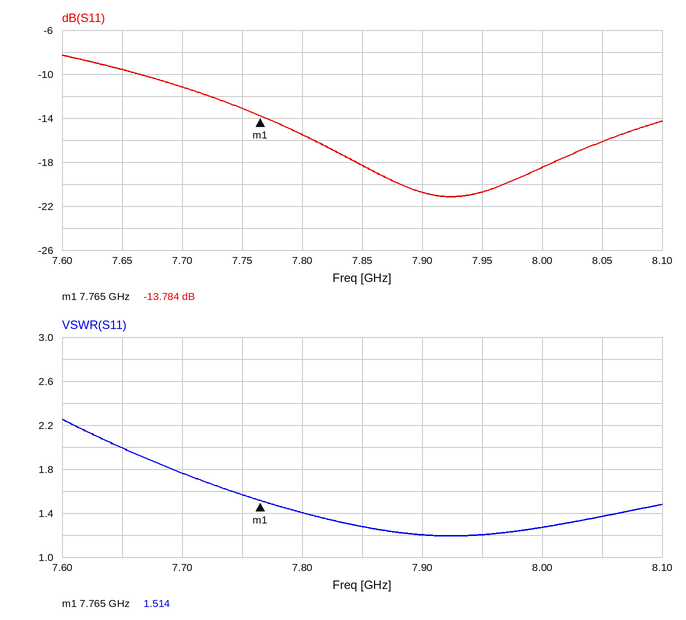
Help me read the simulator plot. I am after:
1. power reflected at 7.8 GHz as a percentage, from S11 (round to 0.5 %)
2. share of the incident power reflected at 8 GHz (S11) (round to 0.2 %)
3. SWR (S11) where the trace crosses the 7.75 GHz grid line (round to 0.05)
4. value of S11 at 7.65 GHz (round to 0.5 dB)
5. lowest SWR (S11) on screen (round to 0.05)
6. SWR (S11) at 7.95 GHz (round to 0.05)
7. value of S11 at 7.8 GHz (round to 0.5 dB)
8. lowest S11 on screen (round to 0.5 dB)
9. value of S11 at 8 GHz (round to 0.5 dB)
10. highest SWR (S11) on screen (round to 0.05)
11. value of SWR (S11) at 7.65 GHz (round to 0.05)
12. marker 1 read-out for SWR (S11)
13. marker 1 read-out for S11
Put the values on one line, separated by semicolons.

3.0 %; 1.4 %; 1.55; -9.5 dB; 1.20; 1.20; -15.5 dB; -21.0 dB; -18.5 dB; 2.25; 2.00; 1.514; -13.784 dB
